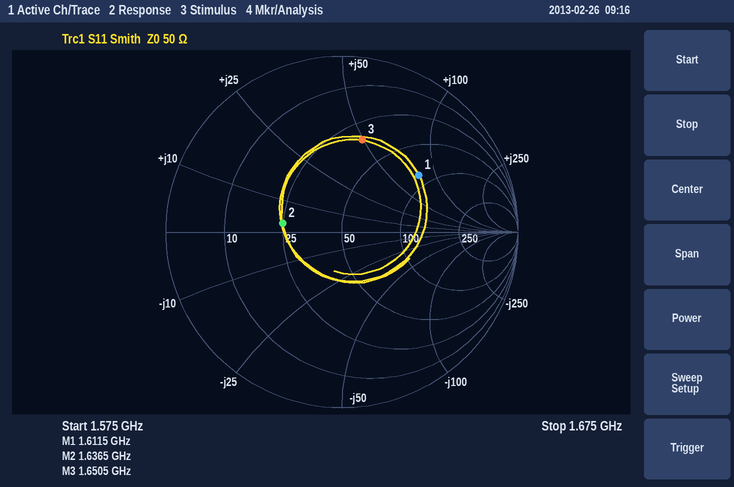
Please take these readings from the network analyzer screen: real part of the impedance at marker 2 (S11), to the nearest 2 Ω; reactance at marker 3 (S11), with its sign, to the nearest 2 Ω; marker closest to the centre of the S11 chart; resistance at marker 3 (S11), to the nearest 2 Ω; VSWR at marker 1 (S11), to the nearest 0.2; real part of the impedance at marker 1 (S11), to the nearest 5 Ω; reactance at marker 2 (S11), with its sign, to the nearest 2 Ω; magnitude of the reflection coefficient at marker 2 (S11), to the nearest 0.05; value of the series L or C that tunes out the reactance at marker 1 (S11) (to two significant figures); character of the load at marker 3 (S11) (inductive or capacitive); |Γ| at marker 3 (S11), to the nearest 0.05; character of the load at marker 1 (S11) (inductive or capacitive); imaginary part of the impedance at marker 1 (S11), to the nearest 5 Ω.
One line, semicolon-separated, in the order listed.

24 Ω; +50 Ω; marker 2; 34 Ω; 3.4; 85 Ω; +2 Ω; 0.35; 1.3 pF; inductive; 0.55; inductive; +75 Ω
